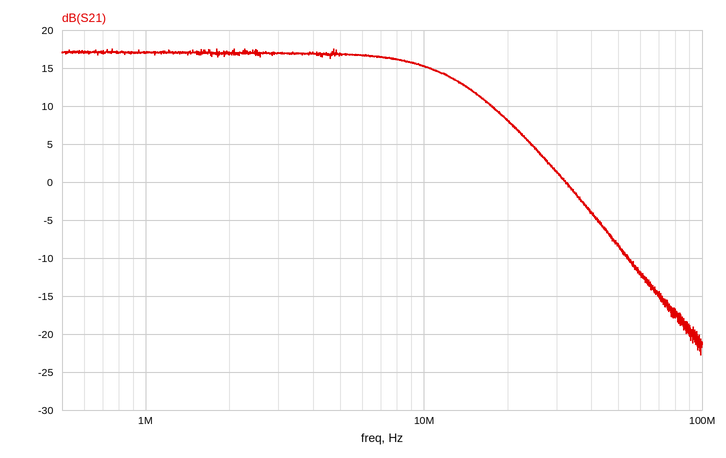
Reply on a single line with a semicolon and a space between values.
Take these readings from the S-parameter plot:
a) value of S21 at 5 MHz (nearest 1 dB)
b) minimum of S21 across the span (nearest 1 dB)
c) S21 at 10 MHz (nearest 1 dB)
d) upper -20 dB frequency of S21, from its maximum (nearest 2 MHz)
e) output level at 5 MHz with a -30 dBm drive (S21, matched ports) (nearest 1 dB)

17 dB; -23 dB; 15 dB; 36 MHz; -13 dBm
